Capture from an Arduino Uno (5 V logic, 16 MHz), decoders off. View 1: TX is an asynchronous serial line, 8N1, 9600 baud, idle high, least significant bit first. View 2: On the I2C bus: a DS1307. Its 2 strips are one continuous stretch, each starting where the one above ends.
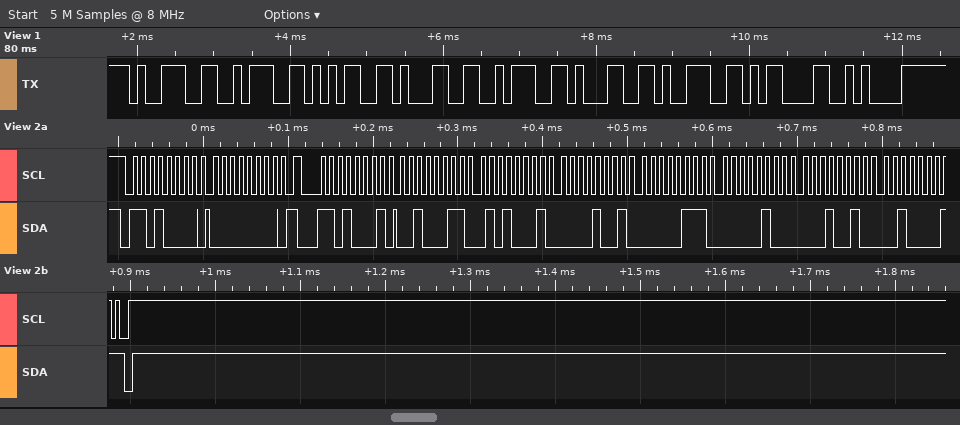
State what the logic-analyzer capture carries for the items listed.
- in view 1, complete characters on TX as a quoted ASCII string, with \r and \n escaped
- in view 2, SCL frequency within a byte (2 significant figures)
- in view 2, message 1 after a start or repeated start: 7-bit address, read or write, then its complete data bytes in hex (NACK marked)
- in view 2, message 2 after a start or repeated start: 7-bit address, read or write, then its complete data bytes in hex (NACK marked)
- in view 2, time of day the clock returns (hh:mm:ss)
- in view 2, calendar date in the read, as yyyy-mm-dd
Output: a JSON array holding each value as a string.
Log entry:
["\"9:51:19\\r\\n\"", "100 kHz", "0x68 write: 00", "0x68 read: 23 51 09 07 04 12 21 NACK", "09:51:23", "2021-12-04"]
